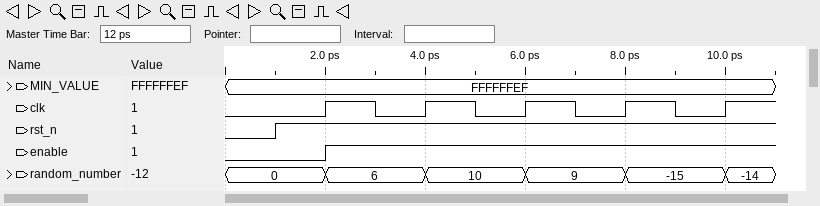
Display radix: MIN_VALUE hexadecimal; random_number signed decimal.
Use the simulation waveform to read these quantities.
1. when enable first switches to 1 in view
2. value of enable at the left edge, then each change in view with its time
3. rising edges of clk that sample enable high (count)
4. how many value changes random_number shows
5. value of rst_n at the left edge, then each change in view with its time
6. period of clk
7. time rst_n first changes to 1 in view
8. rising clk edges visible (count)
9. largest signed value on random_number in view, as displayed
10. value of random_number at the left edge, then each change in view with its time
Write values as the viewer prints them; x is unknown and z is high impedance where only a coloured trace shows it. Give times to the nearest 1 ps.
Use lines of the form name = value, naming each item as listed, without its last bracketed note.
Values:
when enable first switches to 1 in view = 2 ps
value of enable at the left edge, then each change in view with its time = 0, 1 at 2 ps
rising edges of clk that sample enable high = 4
how many value changes random_number shows = 5
value of rst_n at the left edge, then each change in view with its time = 0, 1 at 1 ps
period of clk = 2 ps
time rst_n first changes to 1 in view = 1 ps
rising clk edges visible = 5
largest signed value on random_number in view, as displayed = 10
value of random_number at the left edge, then each change in view with its time = 0, 6 at 2 ps, 10 at 4 ps, 9 at 6 ps, -15 at 8 ps, -14 at 10 ps
